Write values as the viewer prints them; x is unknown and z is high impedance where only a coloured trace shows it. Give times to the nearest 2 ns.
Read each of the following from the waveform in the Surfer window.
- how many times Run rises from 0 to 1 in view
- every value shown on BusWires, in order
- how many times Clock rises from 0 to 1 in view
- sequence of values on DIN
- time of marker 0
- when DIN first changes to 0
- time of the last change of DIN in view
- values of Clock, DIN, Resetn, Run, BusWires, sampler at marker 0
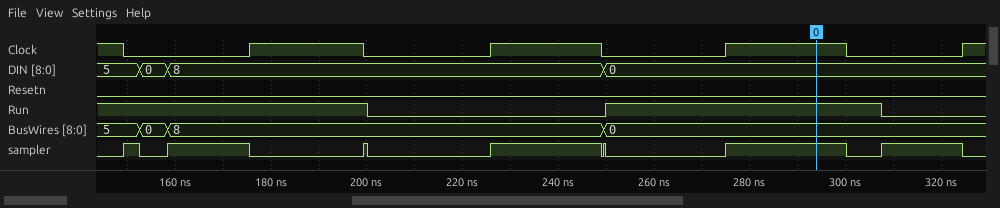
1
5, 0, 8, 0
4
5, 0, 8, 0
294 ns
152 ns
250 ns
Clock=1, DIN=0, Resetn=0, Run=1, BusWires=0, sampler=1
